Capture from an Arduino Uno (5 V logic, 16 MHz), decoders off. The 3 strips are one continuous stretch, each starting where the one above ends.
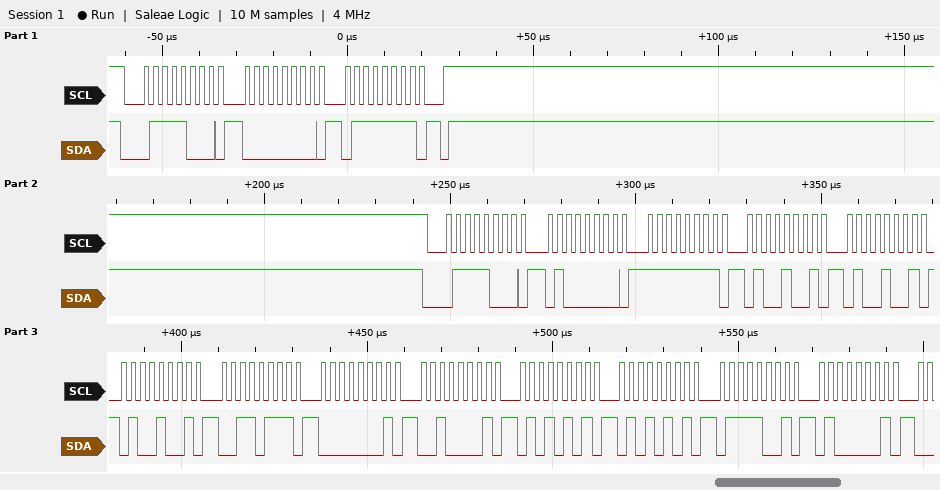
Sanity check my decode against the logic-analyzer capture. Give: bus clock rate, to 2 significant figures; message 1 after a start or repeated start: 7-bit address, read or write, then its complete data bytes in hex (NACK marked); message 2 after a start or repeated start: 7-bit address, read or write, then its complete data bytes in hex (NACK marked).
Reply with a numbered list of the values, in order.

1. 400 kHz
2. 0x3C write: 00 7F
3. 0x3C write: 40 FF 49 49 49 37 01 21 55 55 79 41
